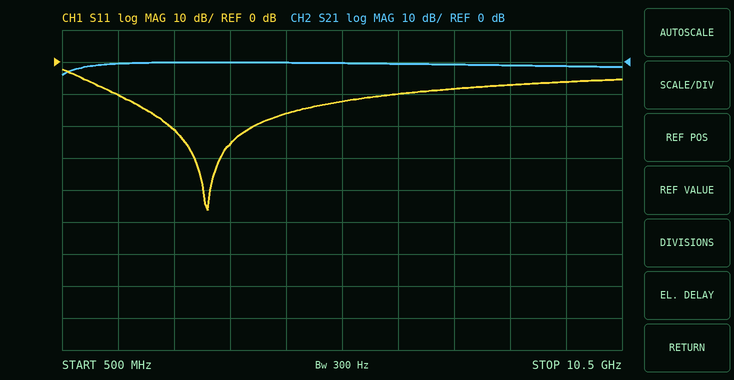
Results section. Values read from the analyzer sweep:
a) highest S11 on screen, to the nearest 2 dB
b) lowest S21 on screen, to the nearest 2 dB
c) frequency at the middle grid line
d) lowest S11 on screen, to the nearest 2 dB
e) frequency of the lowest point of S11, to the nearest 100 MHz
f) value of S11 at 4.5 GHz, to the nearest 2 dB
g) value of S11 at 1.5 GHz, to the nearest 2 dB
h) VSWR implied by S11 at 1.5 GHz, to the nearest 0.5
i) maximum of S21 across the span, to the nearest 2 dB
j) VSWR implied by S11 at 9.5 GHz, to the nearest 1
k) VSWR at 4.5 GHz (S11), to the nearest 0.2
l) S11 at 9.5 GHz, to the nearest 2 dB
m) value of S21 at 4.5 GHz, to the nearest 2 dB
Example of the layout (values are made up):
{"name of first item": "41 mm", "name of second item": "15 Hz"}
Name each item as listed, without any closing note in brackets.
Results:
{"highest S11 on screen, to the nearest 2 dB": "-2 dB", "lowest S21 on screen, to the nearest 2 dB": "-4 dB", "frequency at the middle grid line": "5.5 GHz", "lowest S11 on screen, to the nearest 2 dB": "-46 dB", "frequency of the lowest point of S11, to the nearest 100 MHz": "3.1 GHz", "value of S11 at 4.5 GHz, to the nearest 2 dB": "-16 dB", "value of S11 at 1.5 GHz, to the nearest 2 dB": "-10 dB", "VSWR implied by S11 at 1.5 GHz, to the nearest 0.5": "2.0", "maximum of S21 across the span, to the nearest 2 dB": "0 dB", "VSWR implied by S11 at 9.5 GHz, to the nearest 1": "3", "VSWR at 4.5 GHz (S11), to the nearest 0.2": "1.4", "S11 at 9.5 GHz, to the nearest 2 dB": "-6 dB", "value of S21 at 4.5 GHz, to the nearest 2 dB": "0 dB"}
